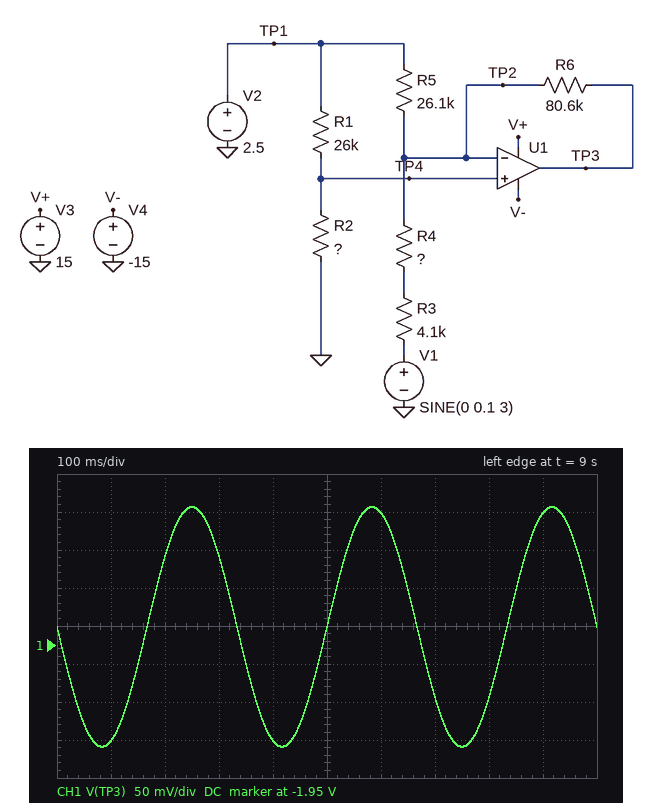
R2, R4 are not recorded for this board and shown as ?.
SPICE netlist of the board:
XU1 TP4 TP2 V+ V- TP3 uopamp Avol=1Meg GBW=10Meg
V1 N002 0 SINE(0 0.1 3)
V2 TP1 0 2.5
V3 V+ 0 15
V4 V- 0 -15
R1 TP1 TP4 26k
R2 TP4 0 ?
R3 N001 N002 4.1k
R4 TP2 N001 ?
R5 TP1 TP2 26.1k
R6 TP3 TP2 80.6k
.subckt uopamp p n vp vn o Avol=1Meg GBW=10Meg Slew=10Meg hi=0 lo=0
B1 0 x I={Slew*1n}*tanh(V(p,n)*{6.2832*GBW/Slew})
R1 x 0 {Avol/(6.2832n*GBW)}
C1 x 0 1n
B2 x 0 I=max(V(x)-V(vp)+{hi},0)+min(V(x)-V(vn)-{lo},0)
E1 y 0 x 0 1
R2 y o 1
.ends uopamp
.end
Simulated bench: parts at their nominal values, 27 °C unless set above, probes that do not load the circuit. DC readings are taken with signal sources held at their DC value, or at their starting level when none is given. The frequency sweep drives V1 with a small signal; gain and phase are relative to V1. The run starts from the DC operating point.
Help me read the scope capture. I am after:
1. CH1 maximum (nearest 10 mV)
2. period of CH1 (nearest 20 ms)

-1.77 V
340 ms
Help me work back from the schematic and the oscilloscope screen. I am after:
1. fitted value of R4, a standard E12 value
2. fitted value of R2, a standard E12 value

47 kΩ
18 kΩ
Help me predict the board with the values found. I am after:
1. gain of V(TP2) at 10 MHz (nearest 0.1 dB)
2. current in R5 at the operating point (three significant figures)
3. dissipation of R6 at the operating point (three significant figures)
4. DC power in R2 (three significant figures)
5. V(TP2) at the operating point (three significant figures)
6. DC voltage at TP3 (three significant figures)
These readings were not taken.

-11.2 dB
56.6 µA
108 µW
58.1 µW
1.02 V
-1.93 V
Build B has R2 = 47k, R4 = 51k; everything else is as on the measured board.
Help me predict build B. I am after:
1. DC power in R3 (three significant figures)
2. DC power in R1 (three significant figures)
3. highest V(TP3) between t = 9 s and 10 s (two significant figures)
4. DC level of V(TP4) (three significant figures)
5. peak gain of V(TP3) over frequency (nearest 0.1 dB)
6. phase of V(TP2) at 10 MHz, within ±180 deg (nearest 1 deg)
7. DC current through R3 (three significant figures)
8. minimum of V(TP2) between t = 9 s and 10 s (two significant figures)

3.50 µW
30.5 µW
1.4 V
1.61 V
3.3 dB
10 deg
29.2 µA
1.6 V
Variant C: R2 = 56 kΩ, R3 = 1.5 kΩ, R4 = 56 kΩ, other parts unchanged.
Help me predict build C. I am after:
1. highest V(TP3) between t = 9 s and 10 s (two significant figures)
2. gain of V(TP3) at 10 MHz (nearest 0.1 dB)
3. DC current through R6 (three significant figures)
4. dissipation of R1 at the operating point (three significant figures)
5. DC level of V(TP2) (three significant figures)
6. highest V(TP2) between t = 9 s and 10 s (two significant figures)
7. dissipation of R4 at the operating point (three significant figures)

1.8 V
-12.0 dB
679 nA
24.2 µW
1.71 V
1.7 V
49.4 µW
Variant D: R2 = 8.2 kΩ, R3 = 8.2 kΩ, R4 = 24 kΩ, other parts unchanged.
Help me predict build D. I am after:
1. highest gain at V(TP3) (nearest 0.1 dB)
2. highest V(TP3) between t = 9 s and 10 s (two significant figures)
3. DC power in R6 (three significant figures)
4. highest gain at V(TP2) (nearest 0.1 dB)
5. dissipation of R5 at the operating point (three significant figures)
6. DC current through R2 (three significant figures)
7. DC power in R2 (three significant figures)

8.0 dB
-3.5 V
237 µW
-8.4 dB
138 µW
73.1 µA
43.8 µW
